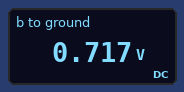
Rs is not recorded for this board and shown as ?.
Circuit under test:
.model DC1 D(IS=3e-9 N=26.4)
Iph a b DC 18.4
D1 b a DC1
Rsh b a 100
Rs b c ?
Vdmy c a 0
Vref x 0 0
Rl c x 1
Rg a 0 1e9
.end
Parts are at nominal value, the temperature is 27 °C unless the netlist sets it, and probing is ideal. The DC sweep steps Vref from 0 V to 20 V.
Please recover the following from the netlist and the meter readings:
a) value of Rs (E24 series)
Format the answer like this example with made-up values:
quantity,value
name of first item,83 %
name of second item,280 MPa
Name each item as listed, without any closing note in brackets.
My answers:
quantity,value
value of Rs,0.039 Ω
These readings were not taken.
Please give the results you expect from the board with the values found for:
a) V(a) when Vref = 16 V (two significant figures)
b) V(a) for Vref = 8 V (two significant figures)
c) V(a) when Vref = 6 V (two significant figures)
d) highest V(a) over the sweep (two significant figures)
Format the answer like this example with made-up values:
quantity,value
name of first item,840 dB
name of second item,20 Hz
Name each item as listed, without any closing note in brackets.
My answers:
quantity,value
V(a) when Vref = 16 V,16 V
V(a) for Vref = 8 V,8.0 V
V(a) when Vref = 6 V,6.0 V
highest V(a) over the sweep,20 V
